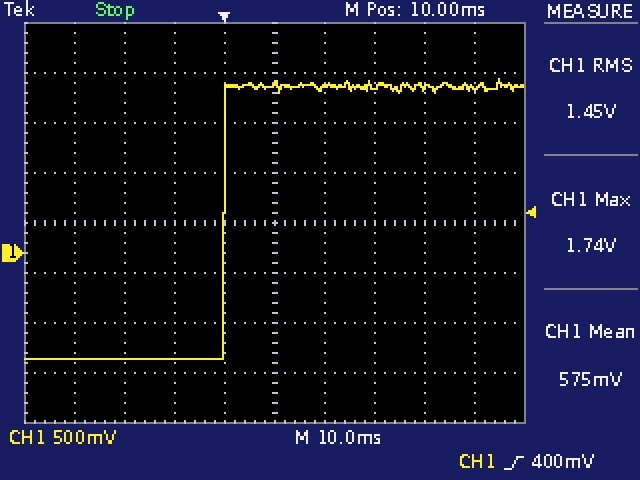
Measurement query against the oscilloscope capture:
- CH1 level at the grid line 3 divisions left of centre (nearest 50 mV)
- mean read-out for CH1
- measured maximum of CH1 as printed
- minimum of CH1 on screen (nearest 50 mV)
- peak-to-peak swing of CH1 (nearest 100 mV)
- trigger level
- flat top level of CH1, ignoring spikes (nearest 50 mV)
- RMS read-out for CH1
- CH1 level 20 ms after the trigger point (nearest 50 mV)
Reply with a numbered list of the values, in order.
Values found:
1. -1.05 V
2. 575 mV
3. 1.74 V
4. -1.05 V
5. 2.80 V
6. 400 mV
7. 1.65 V
8. 1.45 V
9. 1.65 V
